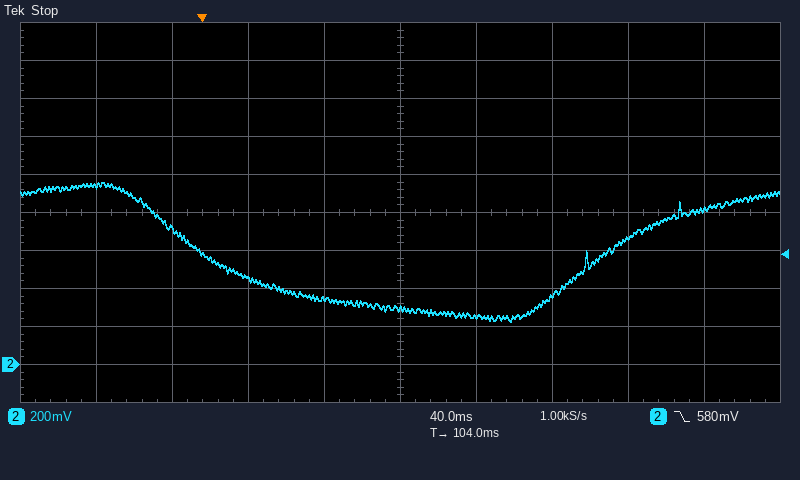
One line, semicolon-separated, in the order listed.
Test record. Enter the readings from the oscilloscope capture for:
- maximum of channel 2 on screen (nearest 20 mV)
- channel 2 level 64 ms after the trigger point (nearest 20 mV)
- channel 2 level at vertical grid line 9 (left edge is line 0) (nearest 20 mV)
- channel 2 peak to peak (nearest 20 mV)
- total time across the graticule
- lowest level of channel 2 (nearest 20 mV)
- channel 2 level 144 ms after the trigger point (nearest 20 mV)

960 mV; 340 mV; 820 mV; 740 mV; 400 ms; 220 mV; 260 mV
